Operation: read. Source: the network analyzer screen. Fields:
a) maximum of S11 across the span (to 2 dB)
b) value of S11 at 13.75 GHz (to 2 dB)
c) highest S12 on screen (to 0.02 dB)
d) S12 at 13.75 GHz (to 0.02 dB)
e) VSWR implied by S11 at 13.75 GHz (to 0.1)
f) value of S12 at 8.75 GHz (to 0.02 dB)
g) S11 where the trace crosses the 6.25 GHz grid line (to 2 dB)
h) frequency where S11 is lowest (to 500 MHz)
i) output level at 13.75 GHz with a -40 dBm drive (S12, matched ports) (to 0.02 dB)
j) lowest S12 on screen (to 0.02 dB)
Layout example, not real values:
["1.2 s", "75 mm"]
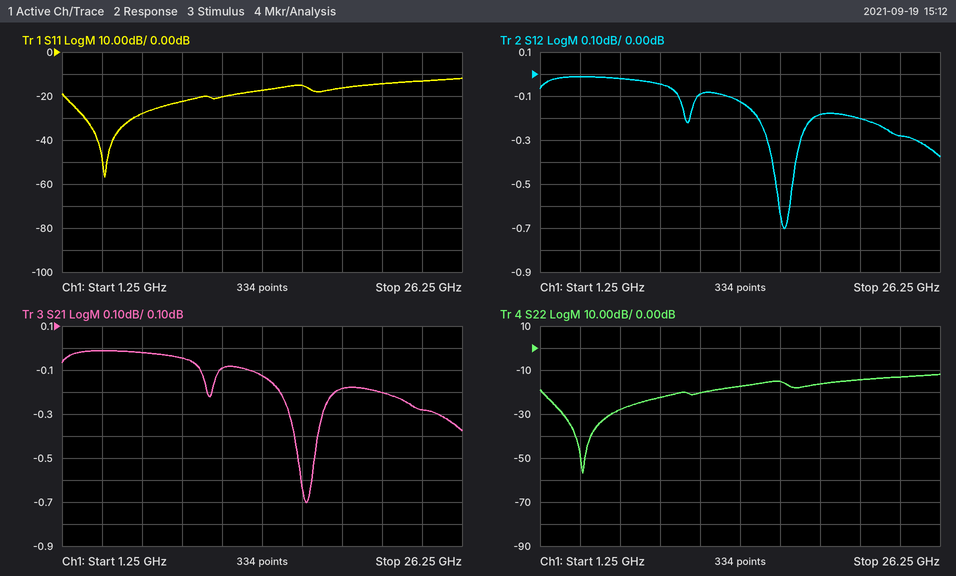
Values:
["-12 dB", "-18 dB", "-0.02 dB", "-0.12 dB", "1.3", "-0.04 dB", "-28 dB", "4.0 GHz", "-40.12 dBm", "-0.70 dB"]
